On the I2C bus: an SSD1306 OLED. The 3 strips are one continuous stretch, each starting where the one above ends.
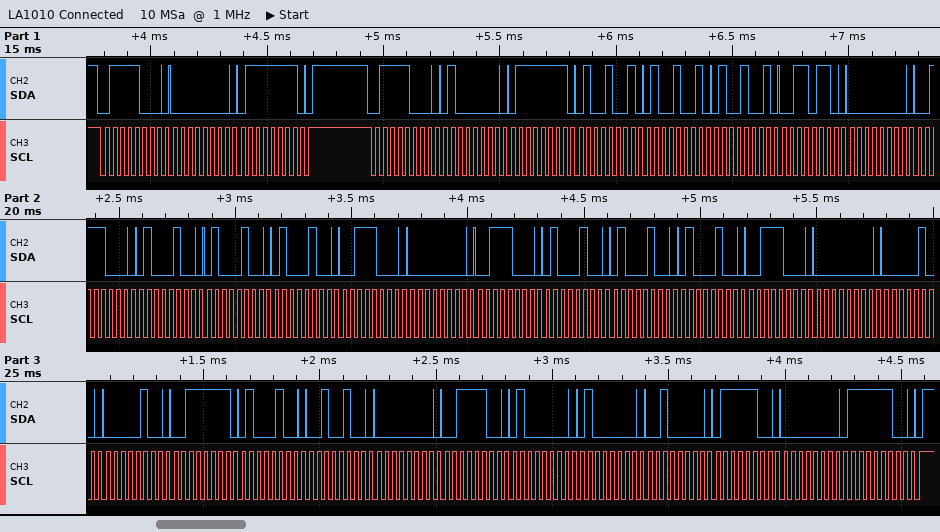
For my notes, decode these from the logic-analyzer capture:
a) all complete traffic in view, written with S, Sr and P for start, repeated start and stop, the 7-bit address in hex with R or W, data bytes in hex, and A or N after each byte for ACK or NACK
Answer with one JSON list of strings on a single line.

["S 3CW A 00 A 7F A P S 3CW A 40 A 7F A 49 A 49 A 49 A 36 A 00 A 38 A 44 A 44 A 44 A 38 A 00 A 38 A 44 A 44 A 44 A 38 A 00 A 04 A 04 A 3F A 44 A 24 A 00 A 3C A 40 A 40 A 20 A 7C A 00 A FC A P"]
